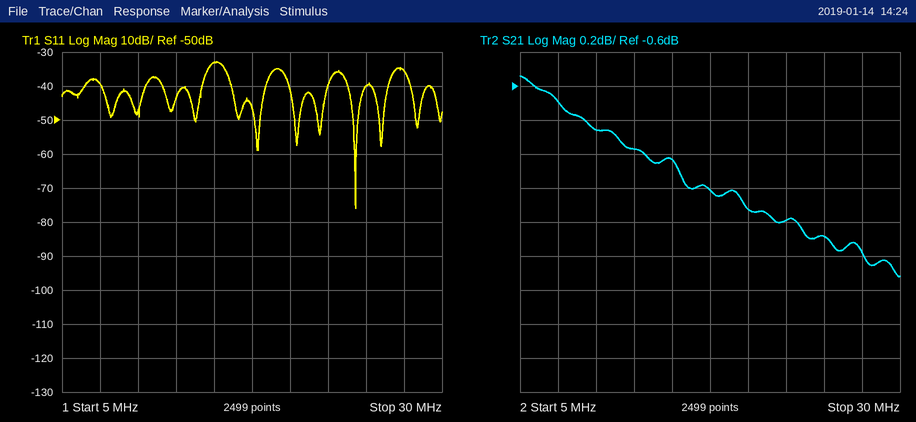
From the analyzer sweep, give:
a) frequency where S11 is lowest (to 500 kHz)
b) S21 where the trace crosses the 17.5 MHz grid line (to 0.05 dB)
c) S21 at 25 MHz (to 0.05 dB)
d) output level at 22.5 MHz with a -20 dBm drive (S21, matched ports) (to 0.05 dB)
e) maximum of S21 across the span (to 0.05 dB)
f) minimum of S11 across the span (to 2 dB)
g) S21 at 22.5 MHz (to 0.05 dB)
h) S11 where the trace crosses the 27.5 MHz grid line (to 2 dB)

24.5 MHz
-1.20 dB
-1.50 dB
-21.40 dBm
-0.55 dB
-76 dB
-1.40 dB
-36 dB
